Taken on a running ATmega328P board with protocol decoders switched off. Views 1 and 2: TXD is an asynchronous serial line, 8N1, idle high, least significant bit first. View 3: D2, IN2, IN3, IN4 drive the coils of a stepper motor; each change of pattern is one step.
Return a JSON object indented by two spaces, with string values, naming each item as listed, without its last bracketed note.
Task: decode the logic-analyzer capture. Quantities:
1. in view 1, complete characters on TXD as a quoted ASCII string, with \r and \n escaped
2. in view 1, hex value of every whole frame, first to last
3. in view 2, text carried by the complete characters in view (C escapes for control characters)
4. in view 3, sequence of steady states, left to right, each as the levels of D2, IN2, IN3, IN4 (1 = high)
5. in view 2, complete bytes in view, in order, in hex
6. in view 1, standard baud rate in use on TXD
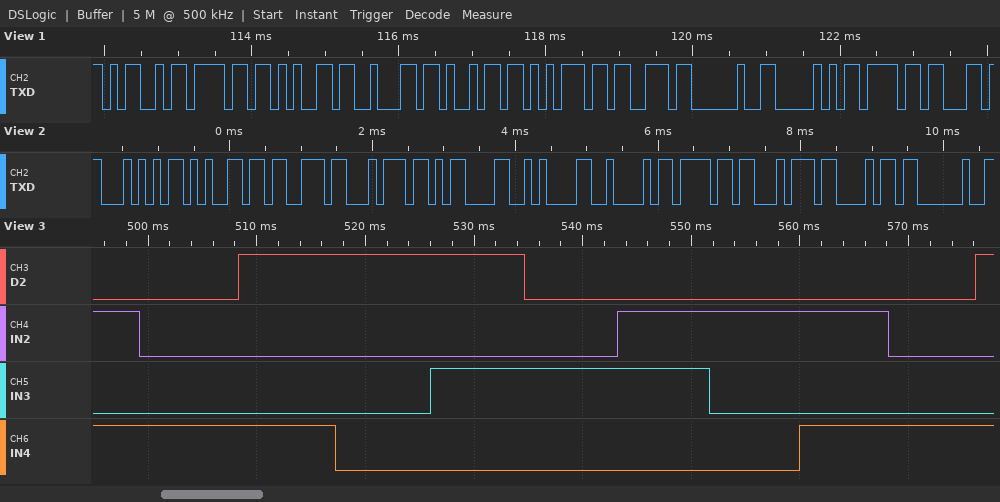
{
  "in view 1, complete characters on TXD as a quoted ASCII string, with \\r and \\n escaped": "\"Moebius Po\"",
  "in view 1, hex value of every whole frame, first to last": "4D 6F 65 62 69 75 73 20 50 6F",
  "in view 2, text carried by the complete characters in view": "\"Test\\r\\nBoth \"",
  "in view 3, sequence of steady states, left to right, each as the levels of D2, IN2, IN3, IN4": "0101 0001 1001 1000 1010 0010 0110 0100 0101 0001 1001",
  "in view 2, complete bytes in view, in order, in hex": "0x54 0x65 0x73 0x74 0x0D 0x0A 0x42 0x6F 0x74 0x68 0x20",
  "in view 1, standard baud rate in use on TXD": "9600 baud"
}
